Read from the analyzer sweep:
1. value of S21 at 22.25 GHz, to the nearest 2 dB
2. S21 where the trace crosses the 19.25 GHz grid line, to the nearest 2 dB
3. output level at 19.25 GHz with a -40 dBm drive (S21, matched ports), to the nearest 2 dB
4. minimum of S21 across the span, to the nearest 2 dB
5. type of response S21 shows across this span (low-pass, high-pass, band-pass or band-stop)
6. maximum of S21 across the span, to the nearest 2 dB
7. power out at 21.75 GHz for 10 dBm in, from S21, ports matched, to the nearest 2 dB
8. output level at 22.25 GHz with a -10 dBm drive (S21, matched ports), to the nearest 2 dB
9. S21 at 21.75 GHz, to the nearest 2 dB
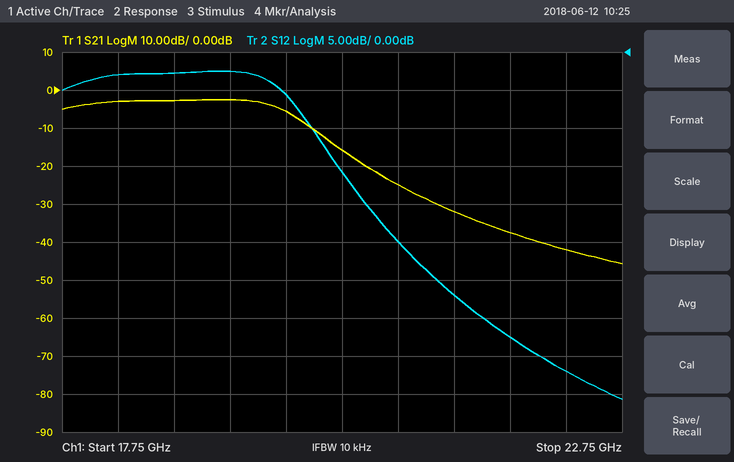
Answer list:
-42 dB
-2 dB
-42 dBm
-46 dB
low-pass
-2 dB
-28 dBm
-52 dBm
-38 dB
